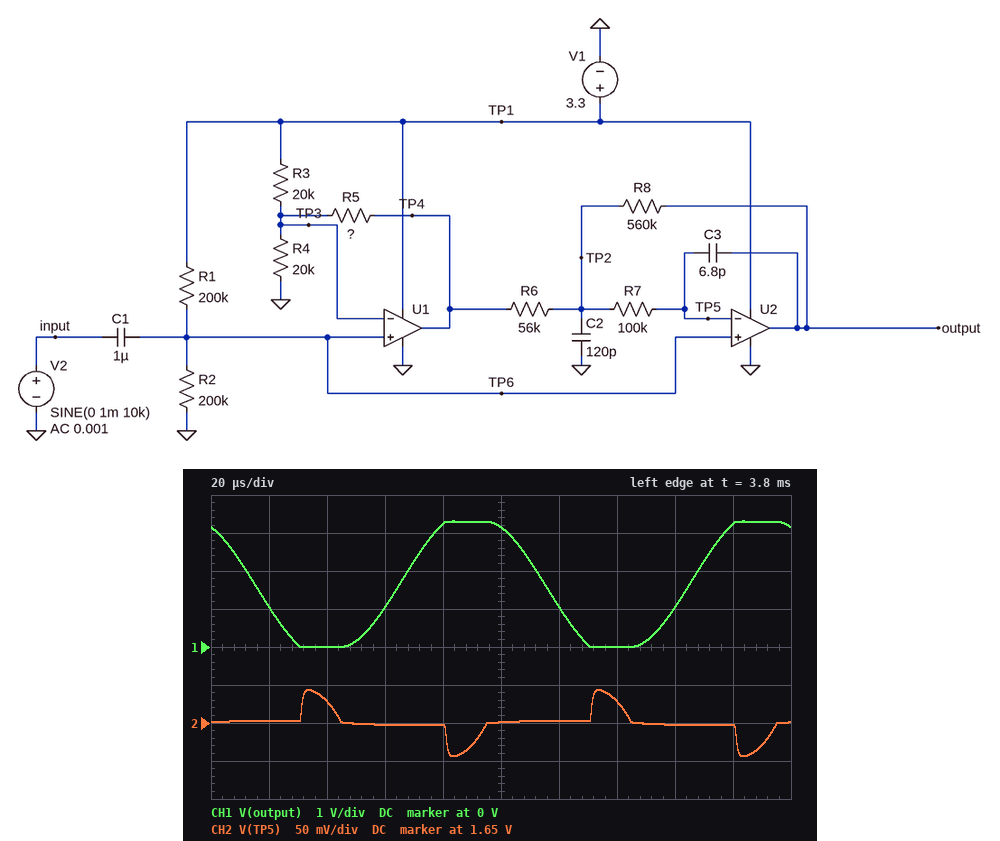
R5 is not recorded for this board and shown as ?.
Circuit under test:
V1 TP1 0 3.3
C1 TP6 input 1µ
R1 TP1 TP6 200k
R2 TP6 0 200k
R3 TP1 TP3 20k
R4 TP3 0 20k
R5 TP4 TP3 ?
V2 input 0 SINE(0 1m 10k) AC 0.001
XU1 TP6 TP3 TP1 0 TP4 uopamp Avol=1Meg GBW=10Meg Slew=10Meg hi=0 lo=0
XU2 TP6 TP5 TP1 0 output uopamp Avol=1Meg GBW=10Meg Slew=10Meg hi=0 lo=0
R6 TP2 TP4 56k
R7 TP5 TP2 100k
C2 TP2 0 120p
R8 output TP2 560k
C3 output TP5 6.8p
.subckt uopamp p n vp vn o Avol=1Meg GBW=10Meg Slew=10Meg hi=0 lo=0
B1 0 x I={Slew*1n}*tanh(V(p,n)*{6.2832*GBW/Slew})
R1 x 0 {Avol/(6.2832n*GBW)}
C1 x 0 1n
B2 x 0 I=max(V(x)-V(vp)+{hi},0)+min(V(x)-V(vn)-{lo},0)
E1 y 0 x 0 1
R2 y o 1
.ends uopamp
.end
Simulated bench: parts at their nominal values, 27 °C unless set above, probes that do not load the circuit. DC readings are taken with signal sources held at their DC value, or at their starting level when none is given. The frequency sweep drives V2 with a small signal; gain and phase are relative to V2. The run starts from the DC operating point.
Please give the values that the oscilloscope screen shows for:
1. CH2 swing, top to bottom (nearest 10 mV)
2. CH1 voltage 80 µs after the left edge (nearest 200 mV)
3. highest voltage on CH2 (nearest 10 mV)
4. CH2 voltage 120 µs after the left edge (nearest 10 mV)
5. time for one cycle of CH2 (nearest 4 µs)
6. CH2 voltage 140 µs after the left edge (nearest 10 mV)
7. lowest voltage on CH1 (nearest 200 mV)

90 mV
3.2 V
1.69 V
1.65 V
100 µs
1.68 V
0 V
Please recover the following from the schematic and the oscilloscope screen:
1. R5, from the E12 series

2.2 MΩ
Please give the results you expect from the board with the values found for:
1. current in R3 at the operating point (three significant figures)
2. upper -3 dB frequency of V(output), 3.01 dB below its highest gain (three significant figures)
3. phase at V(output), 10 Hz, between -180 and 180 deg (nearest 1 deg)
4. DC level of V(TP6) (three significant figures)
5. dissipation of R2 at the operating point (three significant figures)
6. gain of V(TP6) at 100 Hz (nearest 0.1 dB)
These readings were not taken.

82.5 µA
17.3 kHz
-171 deg
1.65 V
13.6 µW
0 dB
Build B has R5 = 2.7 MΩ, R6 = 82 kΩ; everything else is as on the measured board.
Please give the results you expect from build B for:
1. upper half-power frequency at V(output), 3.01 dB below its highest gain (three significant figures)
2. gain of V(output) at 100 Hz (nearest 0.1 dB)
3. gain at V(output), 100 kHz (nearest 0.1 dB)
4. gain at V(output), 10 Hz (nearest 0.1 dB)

21.0 kHz
65.3 dB
31.5 dB
65.2 dB
